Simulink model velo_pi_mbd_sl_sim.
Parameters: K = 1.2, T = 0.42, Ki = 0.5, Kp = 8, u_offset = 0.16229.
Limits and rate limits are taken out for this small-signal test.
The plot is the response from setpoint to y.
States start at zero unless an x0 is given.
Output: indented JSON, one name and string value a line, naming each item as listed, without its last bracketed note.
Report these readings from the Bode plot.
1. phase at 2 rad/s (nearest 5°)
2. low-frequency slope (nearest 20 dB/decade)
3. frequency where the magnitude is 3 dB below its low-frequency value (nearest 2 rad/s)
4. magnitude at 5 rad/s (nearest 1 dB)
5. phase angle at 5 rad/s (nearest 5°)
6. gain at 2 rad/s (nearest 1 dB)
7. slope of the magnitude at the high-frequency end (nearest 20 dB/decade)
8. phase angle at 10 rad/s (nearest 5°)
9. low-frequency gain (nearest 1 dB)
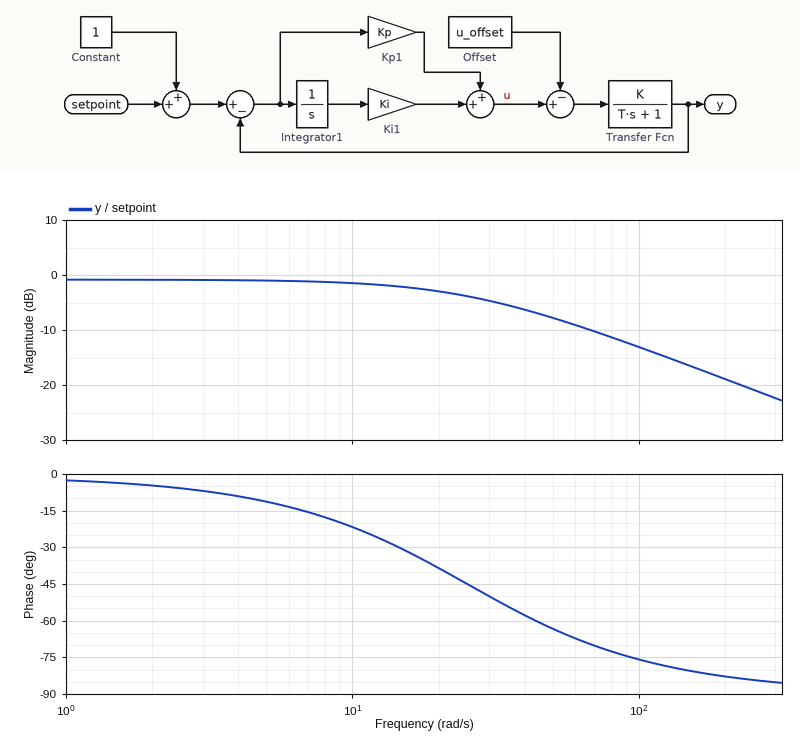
{
  "phase at 2 rad/s": "-5°",
  "low-frequency slope": "0 dB/decade",
  "frequency where the magnitude is 3 dB below its low-frequency value": "26 rad/s",
  "magnitude at 5 rad/s": "-1 dB",
  "phase angle at 5 rad/s": "-10°",
  "gain at 2 rad/s": "-1 dB",
  "slope of the magnitude at the high-frequency end": "-20 dB/decade",
  "phase angle at 10 rad/s": "-20°",
  "low-frequency gain": "-1 dB"
}
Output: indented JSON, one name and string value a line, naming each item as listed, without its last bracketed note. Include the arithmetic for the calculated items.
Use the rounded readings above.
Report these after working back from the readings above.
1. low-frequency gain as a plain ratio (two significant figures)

{
  "low-frequency gain as a plain ratio": "10^(-1 / 20) = 0.89"
}
